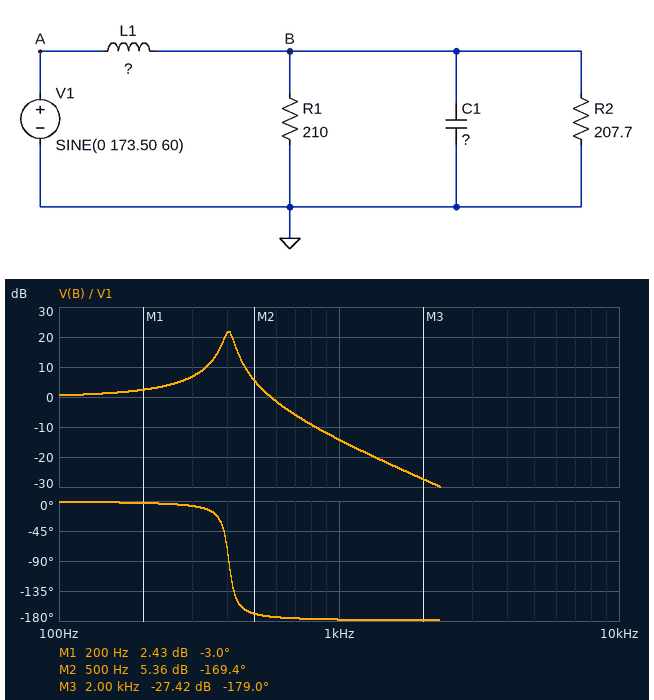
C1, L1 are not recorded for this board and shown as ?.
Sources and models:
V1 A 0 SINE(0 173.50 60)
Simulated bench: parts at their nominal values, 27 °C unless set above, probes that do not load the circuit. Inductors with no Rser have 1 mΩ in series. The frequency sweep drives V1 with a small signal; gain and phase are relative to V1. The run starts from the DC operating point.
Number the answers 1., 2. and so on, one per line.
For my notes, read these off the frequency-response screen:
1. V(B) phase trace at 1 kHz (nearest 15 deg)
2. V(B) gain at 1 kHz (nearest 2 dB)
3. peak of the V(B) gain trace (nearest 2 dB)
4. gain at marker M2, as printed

1. -180 deg
2. -14 dB
3. 22 dB
4. 5.36 dB
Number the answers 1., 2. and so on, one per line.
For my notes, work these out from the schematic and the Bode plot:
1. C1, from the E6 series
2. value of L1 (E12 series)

1. 47 µF
2. 3.3 mH
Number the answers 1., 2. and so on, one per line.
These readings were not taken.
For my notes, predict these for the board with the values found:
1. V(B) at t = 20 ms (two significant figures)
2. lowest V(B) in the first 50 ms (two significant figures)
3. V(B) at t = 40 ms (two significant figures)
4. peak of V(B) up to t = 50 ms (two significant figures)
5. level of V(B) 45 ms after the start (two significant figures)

1. 170 V
2. -180 V
3. 110 V
4. 190 V
5. -170 V
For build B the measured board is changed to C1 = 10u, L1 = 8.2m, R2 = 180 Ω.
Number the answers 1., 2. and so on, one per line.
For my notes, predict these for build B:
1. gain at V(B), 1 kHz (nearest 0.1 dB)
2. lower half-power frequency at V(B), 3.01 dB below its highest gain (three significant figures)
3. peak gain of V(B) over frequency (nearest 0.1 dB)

1. -7.2 dB
2. 453 Hz
3. 10.7 dB
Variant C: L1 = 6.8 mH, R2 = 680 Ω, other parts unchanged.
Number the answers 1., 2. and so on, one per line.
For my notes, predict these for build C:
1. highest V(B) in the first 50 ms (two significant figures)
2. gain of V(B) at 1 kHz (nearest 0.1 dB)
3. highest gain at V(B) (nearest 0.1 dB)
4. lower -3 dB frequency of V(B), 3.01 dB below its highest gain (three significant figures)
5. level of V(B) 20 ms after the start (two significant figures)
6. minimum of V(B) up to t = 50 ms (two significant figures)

1. 190 V
2. -21.3 dB
3. 22.5 dB
4. 270 Hz
5. 180 V
6. -190 V
